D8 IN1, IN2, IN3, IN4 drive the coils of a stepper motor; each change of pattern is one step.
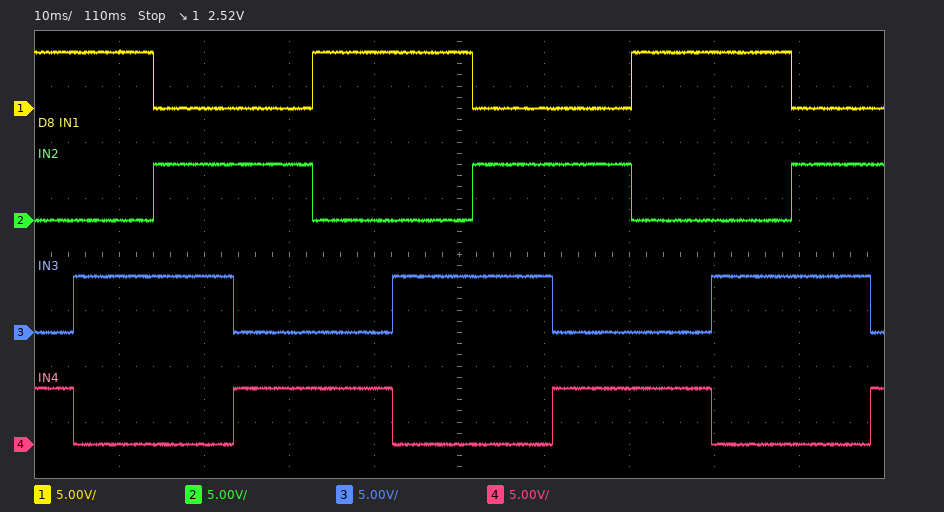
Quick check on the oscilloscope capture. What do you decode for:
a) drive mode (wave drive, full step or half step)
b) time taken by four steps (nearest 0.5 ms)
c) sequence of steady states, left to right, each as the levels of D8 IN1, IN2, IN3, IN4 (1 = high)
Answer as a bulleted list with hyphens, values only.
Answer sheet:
- full step
- 37.5 ms
- 1001 1010 0110 0101 1001 1010 0110 0101 1001 1010 0110 0101
